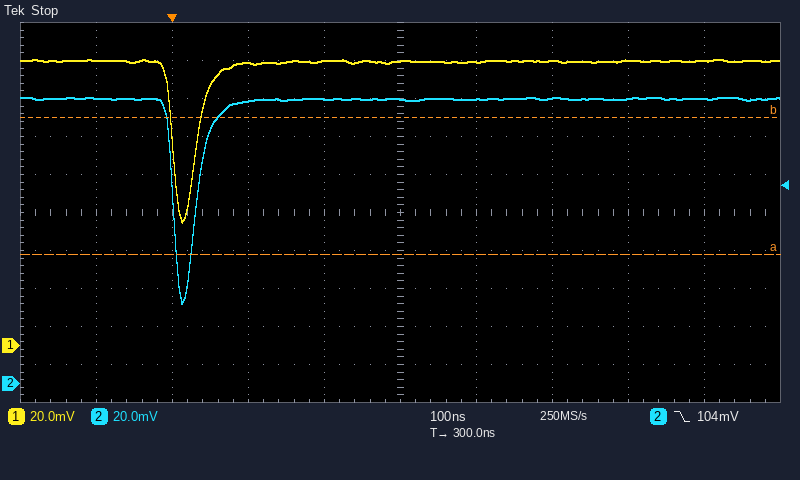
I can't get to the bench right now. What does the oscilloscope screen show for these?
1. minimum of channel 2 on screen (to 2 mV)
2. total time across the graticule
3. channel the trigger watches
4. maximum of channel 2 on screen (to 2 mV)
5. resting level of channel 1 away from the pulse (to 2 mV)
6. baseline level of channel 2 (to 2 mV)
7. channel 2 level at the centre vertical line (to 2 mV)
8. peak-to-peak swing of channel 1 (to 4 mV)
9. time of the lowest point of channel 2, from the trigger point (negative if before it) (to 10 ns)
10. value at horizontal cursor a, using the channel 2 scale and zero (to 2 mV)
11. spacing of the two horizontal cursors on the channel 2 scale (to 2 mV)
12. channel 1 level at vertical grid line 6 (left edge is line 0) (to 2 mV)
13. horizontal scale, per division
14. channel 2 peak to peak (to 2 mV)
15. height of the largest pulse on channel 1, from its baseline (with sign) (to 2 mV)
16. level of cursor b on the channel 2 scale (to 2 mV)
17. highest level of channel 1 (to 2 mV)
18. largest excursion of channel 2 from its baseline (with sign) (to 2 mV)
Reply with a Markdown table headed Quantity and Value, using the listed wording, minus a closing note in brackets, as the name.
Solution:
| Quantity | Value |
|---|---|
| minimum of channel 2 on screen | 42 mV |
| total time across the graticule | 1 µs |
| channel the trigger watches | channel 2 |
| maximum of channel 2 on screen | 150 mV |
| resting level of channel 1 away from the pulse | 150 mV |
| baseline level of channel 2 | 150 mV |
| channel 2 level at the centre vertical line | 150 mV |
| peak-to-peak swing of channel 1 | 84 mV |
| time of the lowest point of channel 2, from the trigger point (negative if before it) | +10 ns |
| value at horizontal cursor a, using the channel 2 scale and zero | 68 mV |
| spacing of the two horizontal cursors on the channel 2 scale | 72 mV |
| channel 1 level at vertical grid line 6 (left edge is line 0) | 150 mV |
| horizontal scale, per division | 100 ns |
| channel 2 peak to peak | 108 mV |
| height of the largest pulse on channel 1, from its baseline (with sign) | -84 mV |
| level of cursor b on the channel 2 scale | 140 mV |
| highest level of channel 1 | 150 mV |
| largest excursion of channel 2 from its baseline (with sign) | -108 mV |
